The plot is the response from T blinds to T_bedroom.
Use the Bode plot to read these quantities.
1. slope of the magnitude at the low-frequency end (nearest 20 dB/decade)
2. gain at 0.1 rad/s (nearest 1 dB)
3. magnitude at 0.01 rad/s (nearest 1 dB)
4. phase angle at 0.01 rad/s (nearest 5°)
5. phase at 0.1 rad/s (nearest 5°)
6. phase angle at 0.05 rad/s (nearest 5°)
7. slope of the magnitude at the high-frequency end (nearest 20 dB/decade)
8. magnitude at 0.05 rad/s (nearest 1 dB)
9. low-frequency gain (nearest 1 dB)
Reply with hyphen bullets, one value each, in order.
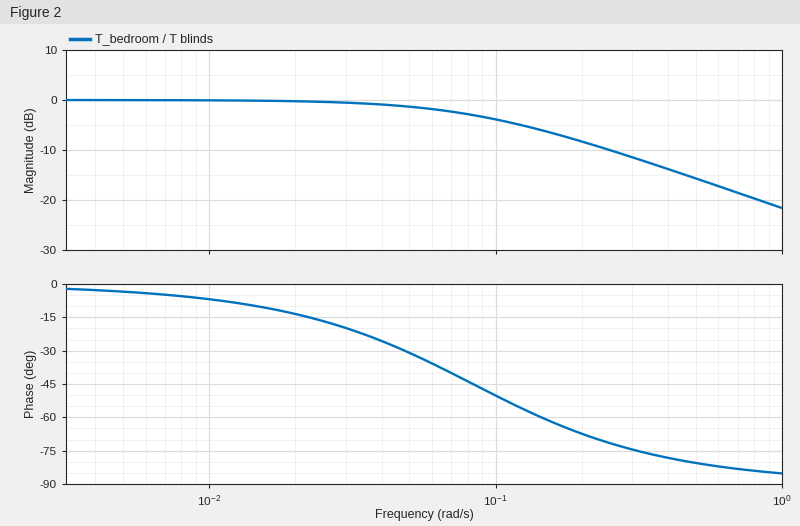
- 0 dB/decade
- -4 dB
- 0 dB
- -5°
- -50°
- -30°
- -20 dB/decade
- -1 dB
- 0 dB
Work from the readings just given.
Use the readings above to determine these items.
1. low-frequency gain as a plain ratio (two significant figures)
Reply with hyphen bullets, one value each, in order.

- 1.0
